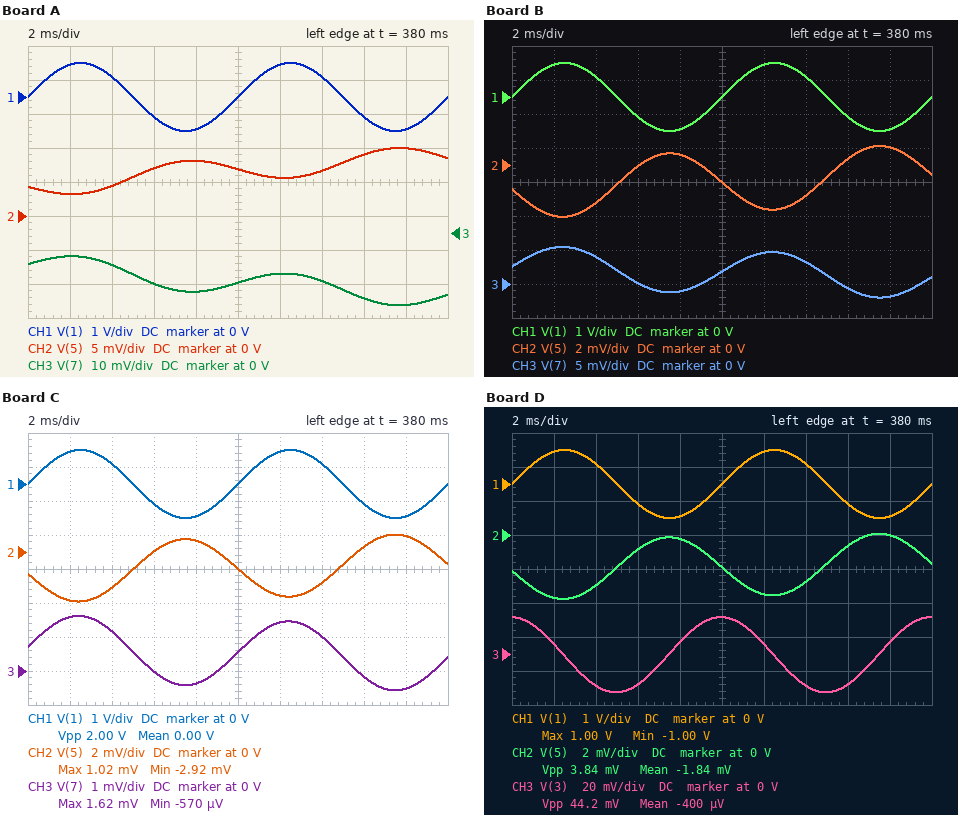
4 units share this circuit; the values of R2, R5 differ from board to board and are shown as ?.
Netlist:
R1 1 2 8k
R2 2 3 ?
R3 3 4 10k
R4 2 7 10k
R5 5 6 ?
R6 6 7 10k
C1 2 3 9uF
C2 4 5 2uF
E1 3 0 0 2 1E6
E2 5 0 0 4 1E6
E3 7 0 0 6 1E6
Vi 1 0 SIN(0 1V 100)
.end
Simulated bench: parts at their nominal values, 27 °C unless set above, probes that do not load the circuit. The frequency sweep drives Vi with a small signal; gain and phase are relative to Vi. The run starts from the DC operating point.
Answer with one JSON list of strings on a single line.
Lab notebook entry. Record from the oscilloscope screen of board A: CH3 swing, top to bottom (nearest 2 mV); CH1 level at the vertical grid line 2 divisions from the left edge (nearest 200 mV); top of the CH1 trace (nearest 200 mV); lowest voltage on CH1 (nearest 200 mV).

["14 mV", "600 mV", "1.0 V", "-1.0 V"]
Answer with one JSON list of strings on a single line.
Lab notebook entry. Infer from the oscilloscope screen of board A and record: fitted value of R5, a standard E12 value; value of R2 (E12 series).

["4.7 kΩ", "18 kΩ"]
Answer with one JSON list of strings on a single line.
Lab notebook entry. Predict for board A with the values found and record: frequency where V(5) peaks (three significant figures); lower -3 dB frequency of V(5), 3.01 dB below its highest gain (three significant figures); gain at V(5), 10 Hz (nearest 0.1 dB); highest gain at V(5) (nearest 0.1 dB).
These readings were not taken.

["5.43 Hz", "4.91 Hz", "-12.1 dB", "10.3 dB"]
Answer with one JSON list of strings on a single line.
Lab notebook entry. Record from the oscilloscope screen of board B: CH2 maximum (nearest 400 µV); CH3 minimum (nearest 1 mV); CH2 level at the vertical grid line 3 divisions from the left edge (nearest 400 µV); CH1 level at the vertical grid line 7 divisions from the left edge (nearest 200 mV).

["1.2 mV", "-2 mV", "0 V", "600 mV"]
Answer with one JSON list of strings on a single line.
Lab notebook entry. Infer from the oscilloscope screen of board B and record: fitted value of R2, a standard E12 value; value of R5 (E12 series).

["6.8 kΩ", "5.6 kΩ"]
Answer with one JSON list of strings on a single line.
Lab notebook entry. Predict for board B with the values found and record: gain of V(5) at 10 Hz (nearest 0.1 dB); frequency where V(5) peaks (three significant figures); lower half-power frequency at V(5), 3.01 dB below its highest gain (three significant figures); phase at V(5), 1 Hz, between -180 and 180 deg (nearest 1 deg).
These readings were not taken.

["-13.1 dB", "4.66 Hz", "3.03 Hz", "-6 deg"]
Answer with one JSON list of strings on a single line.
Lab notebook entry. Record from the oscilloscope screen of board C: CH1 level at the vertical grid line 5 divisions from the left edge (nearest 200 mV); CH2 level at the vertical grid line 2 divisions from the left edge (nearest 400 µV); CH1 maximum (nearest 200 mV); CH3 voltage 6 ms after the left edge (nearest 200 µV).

["0 V", "-2.0 mV", "1.0 V", "0 V"]
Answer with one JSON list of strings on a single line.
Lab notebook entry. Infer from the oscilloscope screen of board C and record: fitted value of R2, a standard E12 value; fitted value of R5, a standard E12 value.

["5.6 kΩ", "18 kΩ"]
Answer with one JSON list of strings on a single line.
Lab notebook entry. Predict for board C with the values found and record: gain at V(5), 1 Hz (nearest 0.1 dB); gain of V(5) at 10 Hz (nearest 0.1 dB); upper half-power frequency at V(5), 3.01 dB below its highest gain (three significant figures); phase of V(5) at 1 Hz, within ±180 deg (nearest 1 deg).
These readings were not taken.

["7.4 dB", "-14.9 dB", "3.18 Hz", "-25 deg"]
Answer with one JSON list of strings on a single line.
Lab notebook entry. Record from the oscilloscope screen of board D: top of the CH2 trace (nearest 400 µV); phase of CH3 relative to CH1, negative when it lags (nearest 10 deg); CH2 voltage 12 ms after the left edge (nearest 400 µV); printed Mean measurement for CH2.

["0 V", "90 deg", "-3.6 mV", "-1.84 mV"]
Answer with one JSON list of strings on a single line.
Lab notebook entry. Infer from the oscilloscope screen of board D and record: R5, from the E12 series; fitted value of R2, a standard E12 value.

["22 kΩ", "5.6 kΩ"]
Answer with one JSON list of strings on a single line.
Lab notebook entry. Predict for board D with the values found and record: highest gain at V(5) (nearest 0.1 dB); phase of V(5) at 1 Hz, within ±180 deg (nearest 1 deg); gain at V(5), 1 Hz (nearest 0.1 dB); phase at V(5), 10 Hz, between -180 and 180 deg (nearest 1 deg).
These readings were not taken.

["9.0 dB", "-30 deg", "9.0 dB", "-161 deg"]
